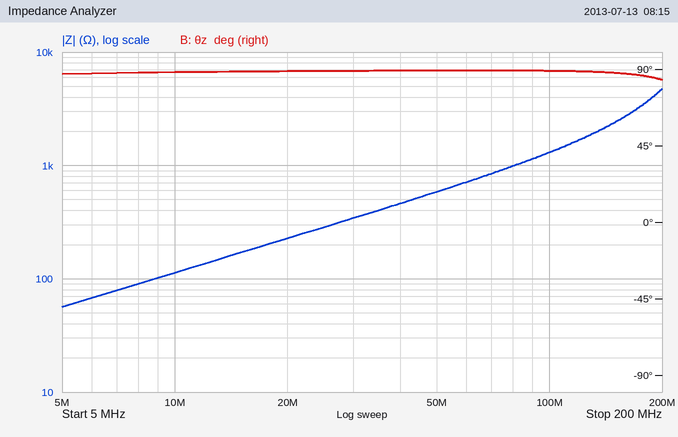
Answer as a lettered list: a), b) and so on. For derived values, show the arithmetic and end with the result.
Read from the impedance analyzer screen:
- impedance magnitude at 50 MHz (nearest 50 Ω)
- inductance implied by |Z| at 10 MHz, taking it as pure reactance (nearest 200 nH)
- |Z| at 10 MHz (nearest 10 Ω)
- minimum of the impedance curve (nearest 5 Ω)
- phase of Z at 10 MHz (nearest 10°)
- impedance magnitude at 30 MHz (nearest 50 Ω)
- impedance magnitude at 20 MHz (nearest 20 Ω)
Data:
a) 600 Ω
b) L = 110 Ω/(2π × 10 MHz) ≈ 1.8 µH
c) 110 Ω
d) 55 Ω
e) 90°
f) 350 Ω
g) 220 Ω
